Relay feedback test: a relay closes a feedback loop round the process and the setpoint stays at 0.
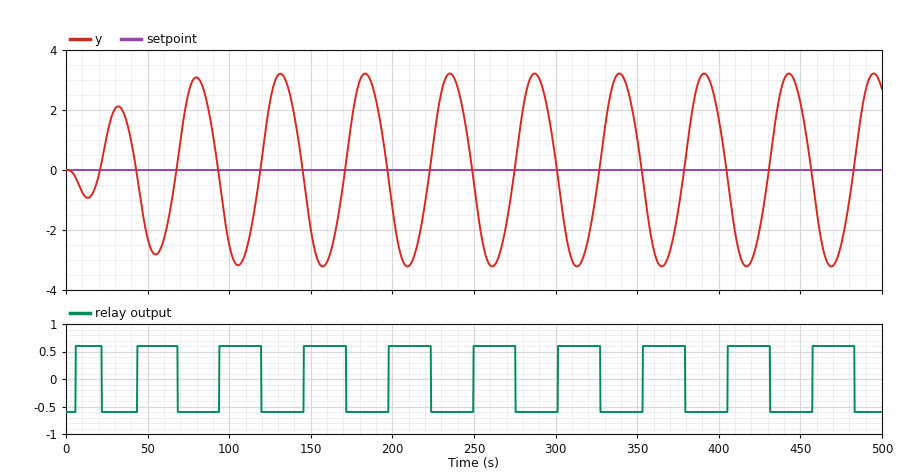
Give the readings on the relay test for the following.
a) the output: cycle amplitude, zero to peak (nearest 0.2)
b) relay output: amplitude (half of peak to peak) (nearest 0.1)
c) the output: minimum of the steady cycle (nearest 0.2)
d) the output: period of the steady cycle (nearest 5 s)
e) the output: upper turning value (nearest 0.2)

3.2
0.6
-3.2
50 s
3.2
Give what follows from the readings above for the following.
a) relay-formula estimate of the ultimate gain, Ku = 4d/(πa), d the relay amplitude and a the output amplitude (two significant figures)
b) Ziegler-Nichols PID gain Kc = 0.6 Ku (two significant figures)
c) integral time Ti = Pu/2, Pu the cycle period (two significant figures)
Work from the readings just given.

0.24
0.14
25 s
